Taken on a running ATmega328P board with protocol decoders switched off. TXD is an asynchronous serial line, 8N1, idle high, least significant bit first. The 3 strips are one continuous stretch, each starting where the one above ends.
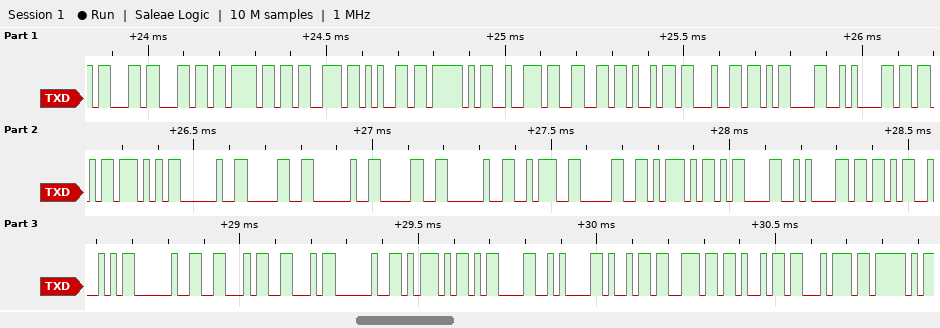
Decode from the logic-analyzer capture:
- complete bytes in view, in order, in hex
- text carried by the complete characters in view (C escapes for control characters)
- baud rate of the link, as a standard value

63 6C 6F 73 65 5F 72 66 69 64 0D 0A 5B 57 20 30 20 30 20 3A 30 5D 0D 0A 5B 52 20 46 46 20 5D 0D 0A 69 6E 69 74 5F
"close_rfid\r\n[W 0 0 :0]\r\n[R FF ]\r\ninit_"
57600 baud
